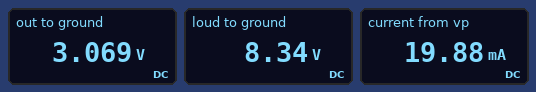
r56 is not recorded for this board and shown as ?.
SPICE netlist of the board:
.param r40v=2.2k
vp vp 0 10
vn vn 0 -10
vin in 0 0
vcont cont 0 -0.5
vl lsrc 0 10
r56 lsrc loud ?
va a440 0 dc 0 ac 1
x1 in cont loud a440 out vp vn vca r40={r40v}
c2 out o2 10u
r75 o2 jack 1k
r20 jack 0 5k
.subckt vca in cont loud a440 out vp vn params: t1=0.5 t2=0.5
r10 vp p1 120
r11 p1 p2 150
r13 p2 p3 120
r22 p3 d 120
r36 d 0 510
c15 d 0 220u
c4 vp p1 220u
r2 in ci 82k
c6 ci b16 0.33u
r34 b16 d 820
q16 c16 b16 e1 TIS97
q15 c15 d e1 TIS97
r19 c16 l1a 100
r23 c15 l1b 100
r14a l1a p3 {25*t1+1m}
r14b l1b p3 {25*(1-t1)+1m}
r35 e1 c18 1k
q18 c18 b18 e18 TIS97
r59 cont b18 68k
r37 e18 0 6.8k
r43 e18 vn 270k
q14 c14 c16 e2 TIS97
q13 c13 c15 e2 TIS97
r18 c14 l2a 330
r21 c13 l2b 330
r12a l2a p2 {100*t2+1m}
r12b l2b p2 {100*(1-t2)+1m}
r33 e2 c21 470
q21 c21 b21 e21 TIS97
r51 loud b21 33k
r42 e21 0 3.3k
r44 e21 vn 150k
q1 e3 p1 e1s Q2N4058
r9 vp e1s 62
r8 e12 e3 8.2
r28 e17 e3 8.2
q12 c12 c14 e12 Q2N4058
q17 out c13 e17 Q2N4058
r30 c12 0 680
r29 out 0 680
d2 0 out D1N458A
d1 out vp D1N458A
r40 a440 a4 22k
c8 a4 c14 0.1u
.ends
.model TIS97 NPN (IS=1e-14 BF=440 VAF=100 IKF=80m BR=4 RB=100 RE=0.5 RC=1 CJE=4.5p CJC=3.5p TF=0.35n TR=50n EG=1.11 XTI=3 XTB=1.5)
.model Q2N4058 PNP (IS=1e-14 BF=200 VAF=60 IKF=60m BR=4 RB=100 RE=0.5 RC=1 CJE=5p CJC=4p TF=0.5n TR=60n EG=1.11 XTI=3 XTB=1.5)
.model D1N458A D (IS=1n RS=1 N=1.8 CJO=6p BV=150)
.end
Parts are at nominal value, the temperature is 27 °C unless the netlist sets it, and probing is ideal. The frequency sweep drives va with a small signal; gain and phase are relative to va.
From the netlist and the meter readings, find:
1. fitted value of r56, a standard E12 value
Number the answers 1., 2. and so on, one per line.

1. 18 kΩ
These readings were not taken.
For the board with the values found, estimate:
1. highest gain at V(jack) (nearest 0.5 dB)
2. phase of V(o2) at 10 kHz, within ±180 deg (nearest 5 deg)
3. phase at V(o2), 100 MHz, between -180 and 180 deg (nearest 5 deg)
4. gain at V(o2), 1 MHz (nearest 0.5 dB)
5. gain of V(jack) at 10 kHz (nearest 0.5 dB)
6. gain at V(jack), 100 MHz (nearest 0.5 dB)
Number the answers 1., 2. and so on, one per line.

1. -12.5 dB
2. 0 deg
3. -135 deg
4. -11.5 dB
5. -12.5 dB
6. -55.5 dB
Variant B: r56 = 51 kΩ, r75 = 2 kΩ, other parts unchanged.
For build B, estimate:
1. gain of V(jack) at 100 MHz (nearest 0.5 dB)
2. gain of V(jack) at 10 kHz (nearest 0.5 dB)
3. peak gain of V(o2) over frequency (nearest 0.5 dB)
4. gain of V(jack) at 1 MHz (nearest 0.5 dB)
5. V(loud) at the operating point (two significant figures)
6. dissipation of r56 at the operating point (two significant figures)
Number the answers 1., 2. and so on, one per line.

1. -57.0 dB
2. -13.5 dB
3. -10.5 dB
4. -14.0 dB
5. 7.1 V
6. 160 µW
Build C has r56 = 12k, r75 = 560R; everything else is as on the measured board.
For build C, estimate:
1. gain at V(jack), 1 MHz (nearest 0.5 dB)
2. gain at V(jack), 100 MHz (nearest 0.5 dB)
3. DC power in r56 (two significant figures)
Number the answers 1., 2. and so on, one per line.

1. -12.5 dB
2. -55.0 dB
3. 130 µW
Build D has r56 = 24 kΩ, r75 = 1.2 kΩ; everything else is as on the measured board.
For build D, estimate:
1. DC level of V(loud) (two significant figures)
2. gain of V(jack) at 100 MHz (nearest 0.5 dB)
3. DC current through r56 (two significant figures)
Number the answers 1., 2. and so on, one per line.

1. 8.0 V
2. -56.0 dB
3. 83 µA
